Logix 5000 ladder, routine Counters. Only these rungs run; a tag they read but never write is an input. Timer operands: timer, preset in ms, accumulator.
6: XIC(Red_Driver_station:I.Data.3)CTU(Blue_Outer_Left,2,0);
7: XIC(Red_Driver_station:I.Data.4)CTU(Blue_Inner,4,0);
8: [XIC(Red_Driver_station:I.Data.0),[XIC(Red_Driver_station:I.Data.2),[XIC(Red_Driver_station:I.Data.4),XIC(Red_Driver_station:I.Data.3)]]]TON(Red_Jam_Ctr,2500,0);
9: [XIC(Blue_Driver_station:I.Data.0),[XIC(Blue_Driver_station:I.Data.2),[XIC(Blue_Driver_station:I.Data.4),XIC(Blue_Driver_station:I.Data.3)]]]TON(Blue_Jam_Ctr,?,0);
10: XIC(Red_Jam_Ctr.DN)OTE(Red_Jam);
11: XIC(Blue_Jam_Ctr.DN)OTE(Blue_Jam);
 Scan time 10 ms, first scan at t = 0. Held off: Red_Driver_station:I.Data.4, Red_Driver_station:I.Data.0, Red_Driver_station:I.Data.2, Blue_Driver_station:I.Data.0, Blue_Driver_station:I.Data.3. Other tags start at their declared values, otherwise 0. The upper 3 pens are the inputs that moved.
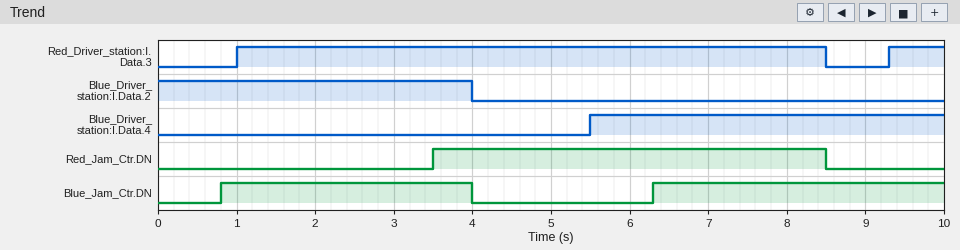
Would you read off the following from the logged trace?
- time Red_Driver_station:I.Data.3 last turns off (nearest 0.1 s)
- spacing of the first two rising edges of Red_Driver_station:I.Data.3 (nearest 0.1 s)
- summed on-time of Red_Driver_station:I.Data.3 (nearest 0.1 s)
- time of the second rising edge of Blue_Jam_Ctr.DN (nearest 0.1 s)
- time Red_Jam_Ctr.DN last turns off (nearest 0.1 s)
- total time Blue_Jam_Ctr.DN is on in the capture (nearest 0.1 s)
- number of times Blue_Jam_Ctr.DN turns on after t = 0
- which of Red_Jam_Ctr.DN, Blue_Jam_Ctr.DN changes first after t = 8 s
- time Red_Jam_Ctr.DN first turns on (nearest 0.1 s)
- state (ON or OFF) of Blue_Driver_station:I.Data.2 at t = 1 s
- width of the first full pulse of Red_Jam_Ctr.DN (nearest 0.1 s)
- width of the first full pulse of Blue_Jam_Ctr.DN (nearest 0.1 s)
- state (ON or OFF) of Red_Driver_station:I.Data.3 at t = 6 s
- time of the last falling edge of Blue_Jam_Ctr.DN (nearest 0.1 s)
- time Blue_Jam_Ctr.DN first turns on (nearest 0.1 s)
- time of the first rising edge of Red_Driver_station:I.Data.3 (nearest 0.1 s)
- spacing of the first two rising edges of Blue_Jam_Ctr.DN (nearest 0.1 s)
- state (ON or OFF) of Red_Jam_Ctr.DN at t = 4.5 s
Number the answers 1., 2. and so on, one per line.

1. 8.5 s
2. 8.3 s
3. 8.2 s
4. 6.3 s
5. 8.5 s
6. 6.9 s
7. 2
8. Red_Jam_Ctr.DN
9. 3.5 s
10. ON
11. 5.0 s
12. 3.2 s
13. ON
14. 4.0 s
15. 0.8 s
16. 1.0 s
17. 5.5 s
18. ON
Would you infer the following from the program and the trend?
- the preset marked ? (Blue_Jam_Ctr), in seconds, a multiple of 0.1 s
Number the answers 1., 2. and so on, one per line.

1. 0.8 s
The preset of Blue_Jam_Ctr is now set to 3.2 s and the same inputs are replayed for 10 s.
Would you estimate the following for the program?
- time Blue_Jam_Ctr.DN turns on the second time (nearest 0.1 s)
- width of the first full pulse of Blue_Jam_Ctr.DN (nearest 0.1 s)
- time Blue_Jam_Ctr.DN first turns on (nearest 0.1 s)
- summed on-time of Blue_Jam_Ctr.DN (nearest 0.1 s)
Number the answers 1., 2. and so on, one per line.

1. 8.7 s
2. 0.8 s
3. 3.2 s
4. 2.1 s
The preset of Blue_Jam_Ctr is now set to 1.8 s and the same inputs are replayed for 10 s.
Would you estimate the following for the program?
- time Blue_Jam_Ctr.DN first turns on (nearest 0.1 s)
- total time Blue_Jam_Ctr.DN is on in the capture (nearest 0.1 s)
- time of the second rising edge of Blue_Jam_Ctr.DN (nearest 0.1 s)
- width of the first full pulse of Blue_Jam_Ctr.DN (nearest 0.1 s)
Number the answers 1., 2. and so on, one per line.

1. 1.8 s
2. 4.9 s
3. 7.3 s
4. 2.2 s
